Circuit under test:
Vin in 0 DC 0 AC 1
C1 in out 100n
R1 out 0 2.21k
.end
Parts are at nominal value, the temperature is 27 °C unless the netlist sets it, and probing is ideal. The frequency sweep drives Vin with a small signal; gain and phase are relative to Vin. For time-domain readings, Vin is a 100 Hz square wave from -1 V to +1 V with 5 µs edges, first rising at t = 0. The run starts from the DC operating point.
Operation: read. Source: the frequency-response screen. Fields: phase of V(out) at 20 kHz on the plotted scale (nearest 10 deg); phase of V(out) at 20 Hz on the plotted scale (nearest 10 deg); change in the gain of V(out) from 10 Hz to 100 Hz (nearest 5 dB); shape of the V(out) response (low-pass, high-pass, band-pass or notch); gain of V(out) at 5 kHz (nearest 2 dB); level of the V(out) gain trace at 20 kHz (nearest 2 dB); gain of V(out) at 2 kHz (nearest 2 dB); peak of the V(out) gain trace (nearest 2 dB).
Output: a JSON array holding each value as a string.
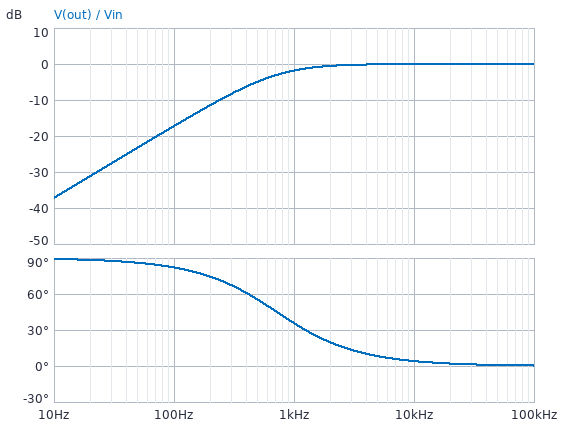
["0 deg", "90 deg", "20 dB", "high-pass", "0 dB", "0 dB", "0 dB", "0 dB"]
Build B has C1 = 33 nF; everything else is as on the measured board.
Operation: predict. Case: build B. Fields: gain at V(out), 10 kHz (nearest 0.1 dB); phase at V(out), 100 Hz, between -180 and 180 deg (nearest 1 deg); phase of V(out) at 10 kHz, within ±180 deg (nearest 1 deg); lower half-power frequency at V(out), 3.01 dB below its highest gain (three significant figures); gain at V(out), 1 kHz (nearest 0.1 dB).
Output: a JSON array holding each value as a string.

["-0.2 dB", "87 deg", "12 deg", "2.18 kHz", "-7.6 dB"]
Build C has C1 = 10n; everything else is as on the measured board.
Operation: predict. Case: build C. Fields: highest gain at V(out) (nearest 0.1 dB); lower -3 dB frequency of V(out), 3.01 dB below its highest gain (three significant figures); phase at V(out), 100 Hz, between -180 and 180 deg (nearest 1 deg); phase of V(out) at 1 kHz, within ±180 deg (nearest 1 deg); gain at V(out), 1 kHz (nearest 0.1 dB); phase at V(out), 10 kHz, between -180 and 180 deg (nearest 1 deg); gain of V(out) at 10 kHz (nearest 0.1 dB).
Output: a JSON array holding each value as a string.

["0 dB", "7.20 kHz", "89 deg", "82 deg", "-17.2 dB", "36 deg", "-1.8 dB"]
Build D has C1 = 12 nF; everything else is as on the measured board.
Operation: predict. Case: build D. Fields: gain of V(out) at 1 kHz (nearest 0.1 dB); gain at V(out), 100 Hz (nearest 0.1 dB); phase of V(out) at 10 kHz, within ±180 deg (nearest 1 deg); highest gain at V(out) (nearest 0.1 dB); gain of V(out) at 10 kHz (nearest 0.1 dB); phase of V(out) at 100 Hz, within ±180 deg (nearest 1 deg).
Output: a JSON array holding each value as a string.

["-15.7 dB", "-35.6 dB", "31 deg", "0 dB", "-1.3 dB", "89 deg"]
